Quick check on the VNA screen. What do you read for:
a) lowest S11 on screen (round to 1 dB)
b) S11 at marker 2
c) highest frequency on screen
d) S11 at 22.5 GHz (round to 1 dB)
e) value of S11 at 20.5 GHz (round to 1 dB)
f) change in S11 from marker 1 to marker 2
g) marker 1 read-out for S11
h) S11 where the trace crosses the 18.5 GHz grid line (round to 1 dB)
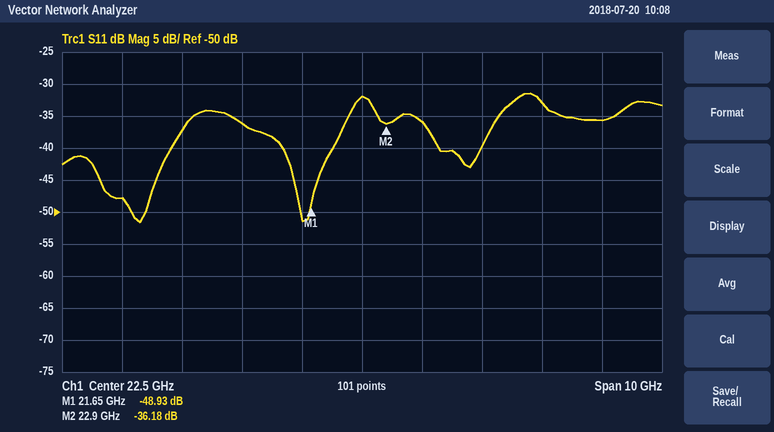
-52 dB
-36.18 dB
27.5 GHz
-32 dB
-36 dB
12.75 dB
-48.93 dB
-48 dB
